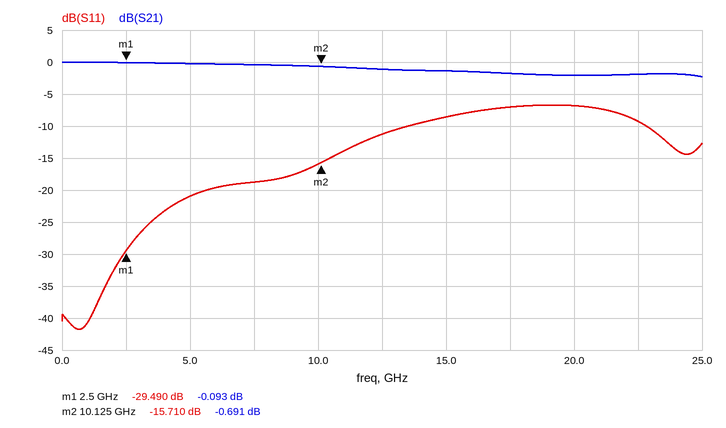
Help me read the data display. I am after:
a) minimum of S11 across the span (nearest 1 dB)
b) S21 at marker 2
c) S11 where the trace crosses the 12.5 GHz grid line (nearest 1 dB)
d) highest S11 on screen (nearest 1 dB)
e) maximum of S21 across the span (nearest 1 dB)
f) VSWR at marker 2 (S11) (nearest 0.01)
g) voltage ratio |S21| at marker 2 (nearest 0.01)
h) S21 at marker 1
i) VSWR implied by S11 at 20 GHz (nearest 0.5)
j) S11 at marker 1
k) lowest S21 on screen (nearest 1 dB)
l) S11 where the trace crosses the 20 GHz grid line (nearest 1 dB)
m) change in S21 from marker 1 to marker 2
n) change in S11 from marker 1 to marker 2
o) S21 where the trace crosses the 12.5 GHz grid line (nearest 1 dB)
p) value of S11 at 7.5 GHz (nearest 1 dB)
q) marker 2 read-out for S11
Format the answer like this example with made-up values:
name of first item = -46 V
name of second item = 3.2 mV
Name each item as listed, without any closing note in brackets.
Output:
minimum of S11 across the span = -42 dB
S21 at marker 2 = -0.691 dB
S11 where the trace crosses the 12.5 GHz grid line = -11 dB
highest S11 on screen = -7 dB
maximum of S21 across the span = 0 dB
VSWR at marker 2 (S11) = 1.39
voltage ratio |S21| at marker 2 = 0.92
S21 at marker 1 = -0.093 dB
VSWR implied by S11 at 20 GHz = 2.5
S11 at marker 1 = -29.490 dB
lowest S21 on screen = -2 dB
S11 where the trace crosses the 20 GHz grid line = -7 dB
change in S21 from marker 1 to marker 2 = -0.598 dB
change in S11 from marker 1 to marker 2 = 13.780 dB
S21 where the trace crosses the 12.5 GHz grid line = -1 dB
value of S11 at 7.5 GHz = -19 dB
marker 2 read-out for S11 = -15.710 dB
